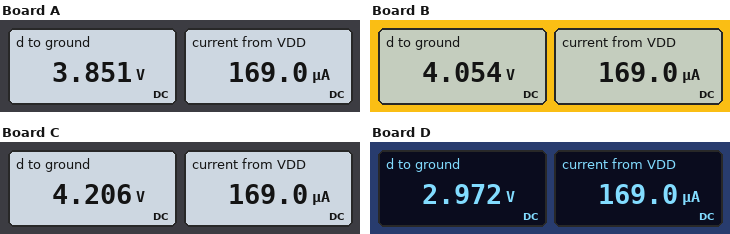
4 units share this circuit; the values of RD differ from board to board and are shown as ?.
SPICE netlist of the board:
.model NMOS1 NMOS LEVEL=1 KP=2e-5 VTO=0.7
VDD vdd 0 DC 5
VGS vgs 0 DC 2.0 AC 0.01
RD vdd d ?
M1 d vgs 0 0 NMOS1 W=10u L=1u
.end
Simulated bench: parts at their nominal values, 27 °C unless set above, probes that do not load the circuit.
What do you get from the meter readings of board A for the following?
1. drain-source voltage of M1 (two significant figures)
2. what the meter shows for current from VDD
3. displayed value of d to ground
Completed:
3.9 V
169.0 µA
3.851 V
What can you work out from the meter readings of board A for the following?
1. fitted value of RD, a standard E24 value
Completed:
6.8 kΩ
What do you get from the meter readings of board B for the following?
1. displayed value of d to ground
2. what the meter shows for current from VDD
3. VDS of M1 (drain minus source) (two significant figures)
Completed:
4.054 V
169.0 µA
4.1 V
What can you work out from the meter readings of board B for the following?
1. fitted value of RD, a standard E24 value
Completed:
5.6 kΩ
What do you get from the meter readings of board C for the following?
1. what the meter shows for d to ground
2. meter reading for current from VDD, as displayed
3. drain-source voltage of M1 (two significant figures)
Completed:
4.206 V
169.0 µA
4.2 V
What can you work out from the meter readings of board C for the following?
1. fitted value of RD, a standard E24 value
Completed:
4.7 kΩ
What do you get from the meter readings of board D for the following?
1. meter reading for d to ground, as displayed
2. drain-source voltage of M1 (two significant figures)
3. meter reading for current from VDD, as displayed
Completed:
2.972 V
3.0 V
169.0 µA
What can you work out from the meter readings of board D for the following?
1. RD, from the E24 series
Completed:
12 kΩ
